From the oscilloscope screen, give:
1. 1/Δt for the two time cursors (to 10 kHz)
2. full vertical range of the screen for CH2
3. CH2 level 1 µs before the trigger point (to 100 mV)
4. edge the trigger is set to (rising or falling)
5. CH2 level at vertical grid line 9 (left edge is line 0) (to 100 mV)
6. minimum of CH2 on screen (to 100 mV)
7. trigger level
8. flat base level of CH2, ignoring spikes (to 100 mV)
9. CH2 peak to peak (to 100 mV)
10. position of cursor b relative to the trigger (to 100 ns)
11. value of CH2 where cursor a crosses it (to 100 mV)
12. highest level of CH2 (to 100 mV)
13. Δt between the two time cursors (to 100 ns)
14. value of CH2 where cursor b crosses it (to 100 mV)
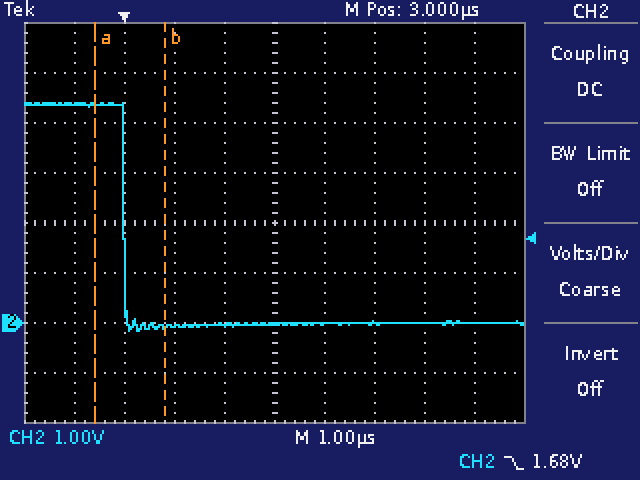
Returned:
710 kHz
8 V
4.4 V
falling
0.0 V
-200 mV
1.68 V
0.0 V
4.6 V
+800 ns
4.4 V
4.4 V
1.4 µs
-100 mV
